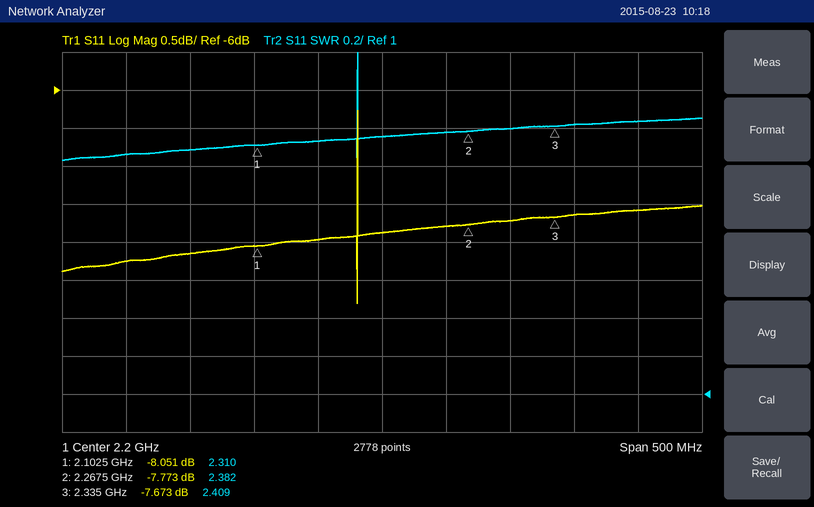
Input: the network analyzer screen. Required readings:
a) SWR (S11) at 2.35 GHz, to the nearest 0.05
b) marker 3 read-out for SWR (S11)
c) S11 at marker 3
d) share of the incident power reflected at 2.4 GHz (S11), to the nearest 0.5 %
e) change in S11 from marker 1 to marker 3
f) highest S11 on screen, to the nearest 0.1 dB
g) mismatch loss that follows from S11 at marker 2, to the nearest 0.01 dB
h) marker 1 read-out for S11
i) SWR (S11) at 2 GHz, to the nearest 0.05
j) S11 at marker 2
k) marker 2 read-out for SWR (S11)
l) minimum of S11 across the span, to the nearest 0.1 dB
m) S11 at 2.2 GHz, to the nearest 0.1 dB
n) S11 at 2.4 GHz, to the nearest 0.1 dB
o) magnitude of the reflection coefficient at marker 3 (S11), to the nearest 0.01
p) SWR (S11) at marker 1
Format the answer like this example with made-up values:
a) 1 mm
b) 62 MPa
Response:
a) 2.40
b) 2.409
c) -7.673 dB
d) 17.5 %
e) 0.378 dB
f) -6.3 dB
g) 0.79 dB
h) -8.051 dB
i) 2.25
j) -7.773 dB
k) 2.382
l) -8.8 dB
m) -7.9 dB
n) -7.6 dB
o) 0.41
p) 2.310
